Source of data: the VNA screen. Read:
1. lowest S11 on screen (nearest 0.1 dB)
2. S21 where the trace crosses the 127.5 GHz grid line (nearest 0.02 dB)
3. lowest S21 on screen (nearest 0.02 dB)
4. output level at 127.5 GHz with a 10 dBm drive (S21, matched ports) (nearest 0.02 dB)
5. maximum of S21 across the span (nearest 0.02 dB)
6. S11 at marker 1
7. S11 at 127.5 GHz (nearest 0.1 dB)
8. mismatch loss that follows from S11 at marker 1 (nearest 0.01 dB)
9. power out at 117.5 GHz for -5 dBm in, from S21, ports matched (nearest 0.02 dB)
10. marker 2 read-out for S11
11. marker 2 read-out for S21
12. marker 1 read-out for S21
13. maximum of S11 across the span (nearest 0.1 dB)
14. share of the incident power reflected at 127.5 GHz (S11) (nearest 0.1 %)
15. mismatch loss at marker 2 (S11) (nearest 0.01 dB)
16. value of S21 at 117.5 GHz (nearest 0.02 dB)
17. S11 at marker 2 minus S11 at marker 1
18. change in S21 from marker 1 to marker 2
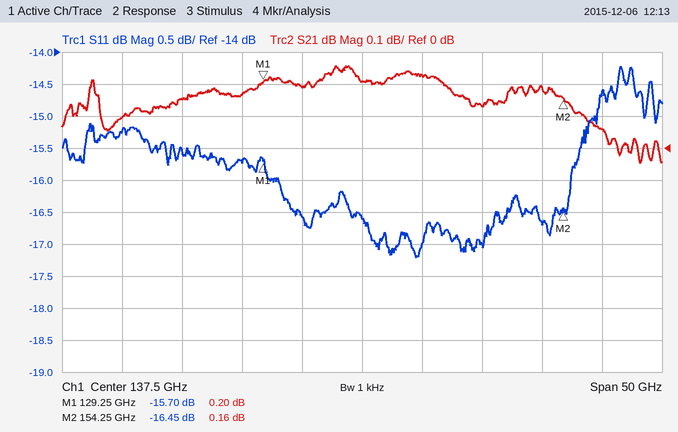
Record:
-17.2 dB
0.16 dB
-0.04 dB
10.16 dBm
0.26 dB
-15.70 dB
-15.7 dB
0.12 dB
-4.90 dBm
-16.45 dB
0.16 dB
0.20 dB
-14.2 dB
2.7 %
0.10 dB
0.10 dB
-0.75 dB
-0.04 dB
